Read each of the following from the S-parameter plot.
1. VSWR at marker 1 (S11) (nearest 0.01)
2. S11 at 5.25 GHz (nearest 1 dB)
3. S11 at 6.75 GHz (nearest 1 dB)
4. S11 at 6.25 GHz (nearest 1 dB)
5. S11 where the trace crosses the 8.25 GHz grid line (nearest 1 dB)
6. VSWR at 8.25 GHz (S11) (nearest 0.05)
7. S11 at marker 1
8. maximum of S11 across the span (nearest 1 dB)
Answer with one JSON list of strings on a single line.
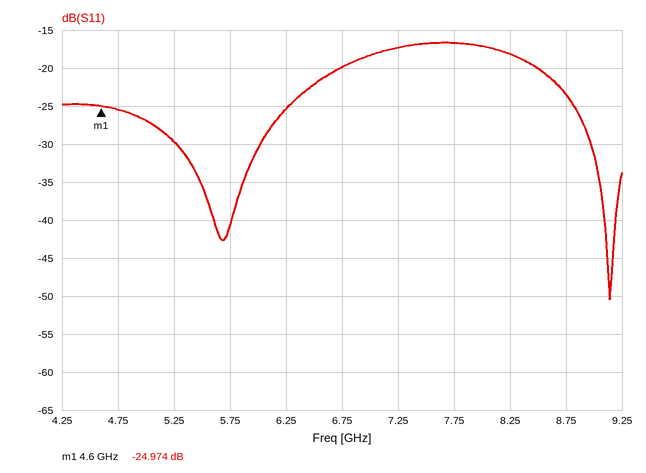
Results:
["1.12", "-30 dB", "-20 dB", "-25 dB", "-18 dB", "1.30", "-24.974 dB", "-17 dB"]
